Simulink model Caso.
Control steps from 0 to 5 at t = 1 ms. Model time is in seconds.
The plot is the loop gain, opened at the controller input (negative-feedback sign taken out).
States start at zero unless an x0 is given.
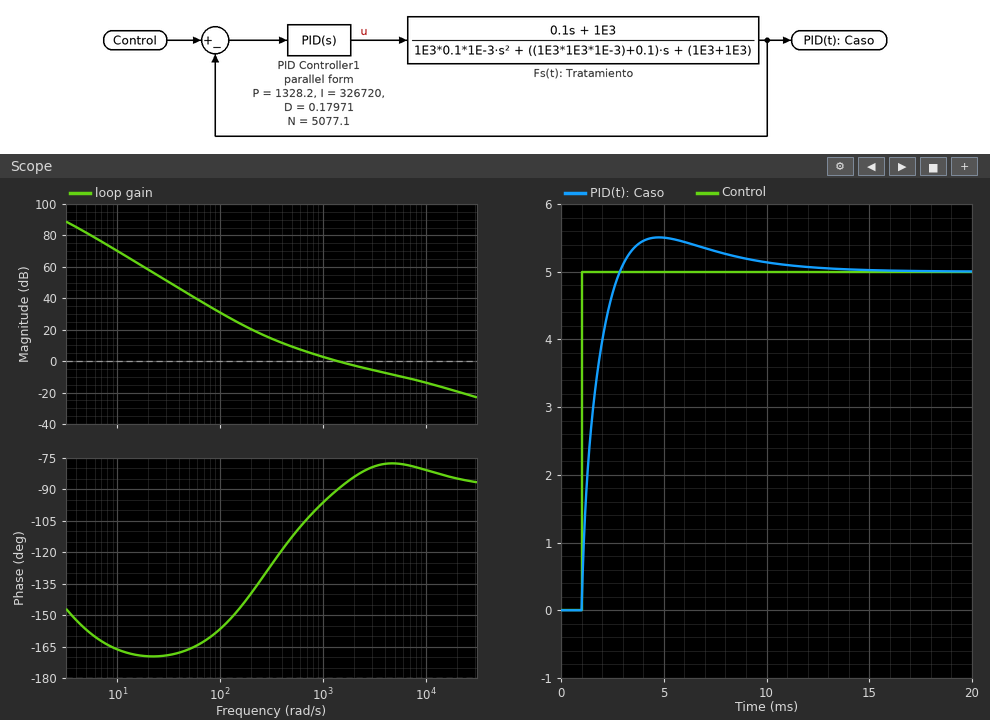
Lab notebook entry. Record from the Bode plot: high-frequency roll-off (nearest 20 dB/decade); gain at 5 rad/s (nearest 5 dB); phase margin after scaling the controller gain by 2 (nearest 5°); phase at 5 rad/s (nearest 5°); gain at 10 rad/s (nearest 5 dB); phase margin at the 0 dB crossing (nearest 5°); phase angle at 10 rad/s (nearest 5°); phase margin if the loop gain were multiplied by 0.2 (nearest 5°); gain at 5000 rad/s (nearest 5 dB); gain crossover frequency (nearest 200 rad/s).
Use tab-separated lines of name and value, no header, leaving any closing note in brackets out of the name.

high-frequency roll-off	-20 dB/decade
gain at 5 rad/s	80 dB
phase margin after scaling the controller gain by 2	100°
phase at 5 rad/s	-155°
gain at 10 rad/s	70 dB
phase margin at the 0 dB crossing	90°
phase angle at 10 rad/s	-165°
phase margin if the loop gain were multiplied by 0.2	55°
gain at 5000 rad/s	-10 dB
gain crossover frequency	1400 rad/s
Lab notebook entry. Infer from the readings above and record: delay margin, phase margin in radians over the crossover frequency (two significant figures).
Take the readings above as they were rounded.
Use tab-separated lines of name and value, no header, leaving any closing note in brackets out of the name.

delay margin, phase margin in radians over the crossover frequency	0.0011 s
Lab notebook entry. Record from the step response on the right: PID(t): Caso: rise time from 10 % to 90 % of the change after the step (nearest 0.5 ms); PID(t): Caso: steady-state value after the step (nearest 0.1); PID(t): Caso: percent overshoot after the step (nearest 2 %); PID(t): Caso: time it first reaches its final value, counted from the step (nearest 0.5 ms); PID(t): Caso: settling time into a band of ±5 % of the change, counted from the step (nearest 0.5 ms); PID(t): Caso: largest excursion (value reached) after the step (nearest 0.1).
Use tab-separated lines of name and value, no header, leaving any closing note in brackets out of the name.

PID(t): Caso: rise time from 10 % to 90 % of the change after the step	1.5 ms
PID(t): Caso: steady-state value after the step	5.0
PID(t): Caso: percent overshoot after the step	10 %
PID(t): Caso: time it first reaches its final value, counted from the step	2.0 ms
PID(t): Caso: settling time into a band of ±5 % of the change, counted from the step	7.0 ms
PID(t): Caso: largest excursion (value reached) after the step	5.5
